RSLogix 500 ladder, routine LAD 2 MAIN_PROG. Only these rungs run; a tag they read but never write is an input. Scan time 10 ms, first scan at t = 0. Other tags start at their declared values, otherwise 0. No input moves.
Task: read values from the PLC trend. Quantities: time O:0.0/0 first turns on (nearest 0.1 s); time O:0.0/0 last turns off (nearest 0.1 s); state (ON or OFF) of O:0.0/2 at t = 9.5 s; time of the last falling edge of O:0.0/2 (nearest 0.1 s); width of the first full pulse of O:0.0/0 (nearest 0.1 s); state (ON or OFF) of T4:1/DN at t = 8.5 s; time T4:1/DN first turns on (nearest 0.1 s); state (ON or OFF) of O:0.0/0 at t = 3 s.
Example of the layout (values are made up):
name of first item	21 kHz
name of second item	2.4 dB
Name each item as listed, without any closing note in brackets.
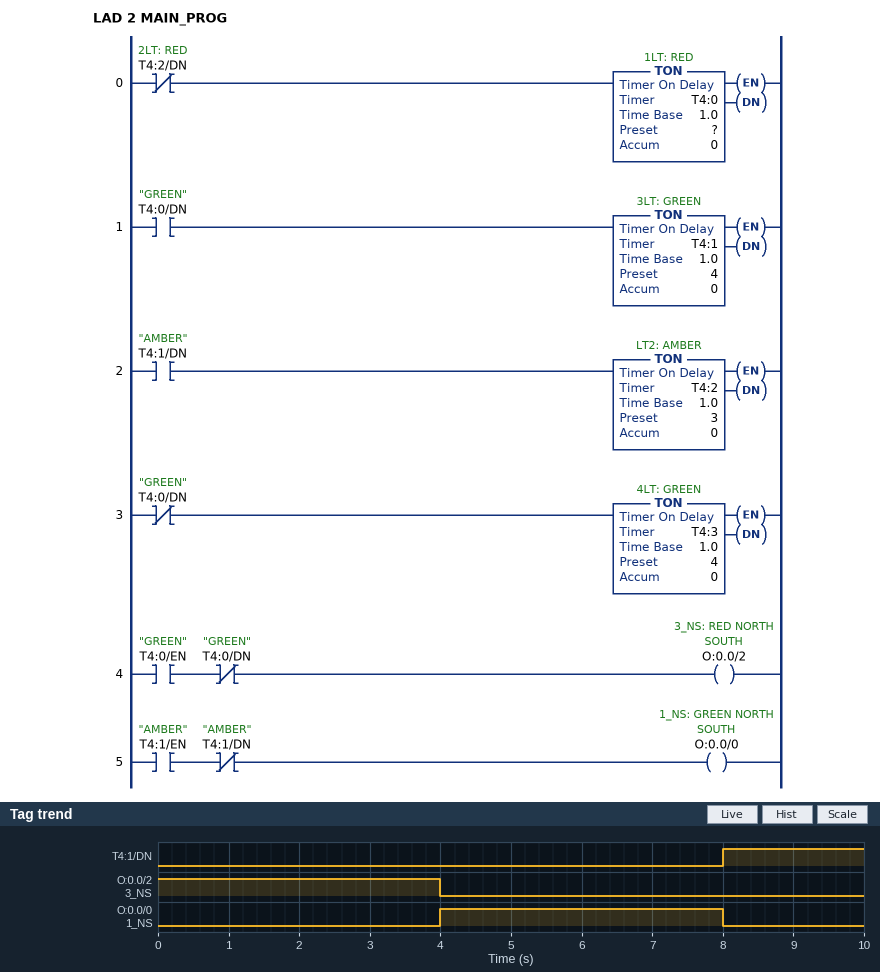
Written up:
time O:0.0/0 first turns on	4.0 s
time O:0.0/0 last turns off	8.0 s
state (ON or OFF) of O:0.0/2 at t = 9.5 s	OFF
time of the last falling edge of O:0.0/2	4.0 s
width of the first full pulse of O:0.0/0	4.0 s
state (ON or OFF) of T4:1/DN at t = 8.5 s	ON
time T4:1/DN first turns on	8.0 s
state (ON or OFF) of O:0.0/0 at t = 3 s	OFF
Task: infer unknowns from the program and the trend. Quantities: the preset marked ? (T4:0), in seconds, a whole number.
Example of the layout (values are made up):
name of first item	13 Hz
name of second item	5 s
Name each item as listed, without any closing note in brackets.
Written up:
the preset marked ? (T4:0), in seconds, a whole number	4 s
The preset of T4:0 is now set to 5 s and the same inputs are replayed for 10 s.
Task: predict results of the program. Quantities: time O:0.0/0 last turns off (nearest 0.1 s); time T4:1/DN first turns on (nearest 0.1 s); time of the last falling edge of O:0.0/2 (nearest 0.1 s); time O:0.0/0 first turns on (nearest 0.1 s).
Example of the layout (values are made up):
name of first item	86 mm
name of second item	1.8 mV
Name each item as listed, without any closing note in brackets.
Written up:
time O:0.0/0 last turns off	9.0 s
time T4:1/DN first turns on	9.0 s
time of the last falling edge of O:0.0/2	5.0 s
time O:0.0/0 first turns on	5.0 s
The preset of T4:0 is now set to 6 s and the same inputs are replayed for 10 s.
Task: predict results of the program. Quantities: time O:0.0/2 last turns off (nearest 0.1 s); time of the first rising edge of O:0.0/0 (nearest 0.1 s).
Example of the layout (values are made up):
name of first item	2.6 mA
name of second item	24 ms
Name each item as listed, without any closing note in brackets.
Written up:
time O:0.0/2 last turns off	6.0 s
time of the first rising edge of O:0.0/0	6.0 s
